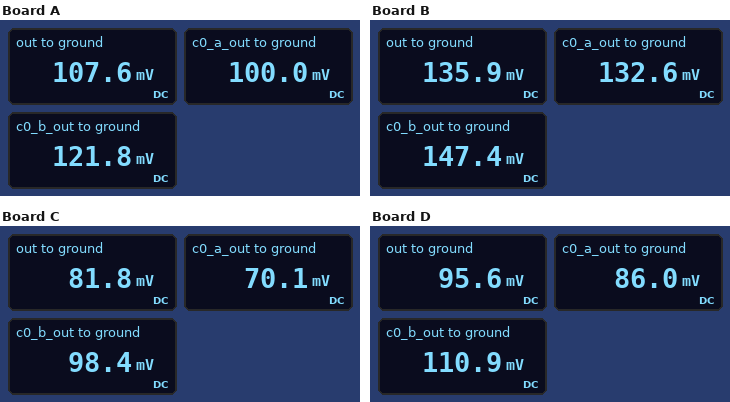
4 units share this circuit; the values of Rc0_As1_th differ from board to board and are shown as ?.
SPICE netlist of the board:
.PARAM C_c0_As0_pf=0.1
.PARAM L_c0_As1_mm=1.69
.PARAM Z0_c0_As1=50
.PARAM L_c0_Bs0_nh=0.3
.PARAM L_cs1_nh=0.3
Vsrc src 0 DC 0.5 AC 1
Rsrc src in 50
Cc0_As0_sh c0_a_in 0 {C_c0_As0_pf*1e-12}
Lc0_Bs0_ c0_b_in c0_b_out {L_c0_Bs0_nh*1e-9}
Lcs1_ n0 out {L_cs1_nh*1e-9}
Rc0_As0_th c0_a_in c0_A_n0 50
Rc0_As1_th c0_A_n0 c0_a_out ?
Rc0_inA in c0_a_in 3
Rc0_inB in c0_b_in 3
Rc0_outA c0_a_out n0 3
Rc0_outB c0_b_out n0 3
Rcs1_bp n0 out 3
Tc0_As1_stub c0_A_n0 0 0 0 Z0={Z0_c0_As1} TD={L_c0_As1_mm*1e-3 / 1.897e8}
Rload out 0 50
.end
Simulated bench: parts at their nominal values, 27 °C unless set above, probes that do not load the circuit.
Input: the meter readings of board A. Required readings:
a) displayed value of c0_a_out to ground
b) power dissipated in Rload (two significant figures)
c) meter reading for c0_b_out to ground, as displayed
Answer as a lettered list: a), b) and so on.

a) 100.0 mV
b) 230 µW
c) 121.8 mV
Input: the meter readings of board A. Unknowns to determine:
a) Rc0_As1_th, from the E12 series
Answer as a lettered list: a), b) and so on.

a) 39 Ω
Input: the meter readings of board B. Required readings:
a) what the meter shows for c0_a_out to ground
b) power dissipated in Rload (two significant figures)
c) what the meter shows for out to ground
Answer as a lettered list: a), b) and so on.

a) 132.6 mV
b) 370 µW
c) 135.9 mV
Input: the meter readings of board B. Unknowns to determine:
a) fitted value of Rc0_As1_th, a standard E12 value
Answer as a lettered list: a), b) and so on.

a) 120 Ω
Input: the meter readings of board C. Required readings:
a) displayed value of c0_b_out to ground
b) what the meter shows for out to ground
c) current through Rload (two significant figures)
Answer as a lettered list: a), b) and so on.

a) 98.4 mV
b) 81.8 mV
c) 1.6 mA
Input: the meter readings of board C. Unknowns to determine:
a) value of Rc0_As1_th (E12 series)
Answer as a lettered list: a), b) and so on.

a) 18 Ω
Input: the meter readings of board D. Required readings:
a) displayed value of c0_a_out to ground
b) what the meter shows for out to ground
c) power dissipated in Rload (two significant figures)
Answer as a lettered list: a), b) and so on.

a) 86.0 mV
b) 95.6 mV
c) 180 µW
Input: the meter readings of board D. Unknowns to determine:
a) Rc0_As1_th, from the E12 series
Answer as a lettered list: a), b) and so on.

a) 27 Ω
